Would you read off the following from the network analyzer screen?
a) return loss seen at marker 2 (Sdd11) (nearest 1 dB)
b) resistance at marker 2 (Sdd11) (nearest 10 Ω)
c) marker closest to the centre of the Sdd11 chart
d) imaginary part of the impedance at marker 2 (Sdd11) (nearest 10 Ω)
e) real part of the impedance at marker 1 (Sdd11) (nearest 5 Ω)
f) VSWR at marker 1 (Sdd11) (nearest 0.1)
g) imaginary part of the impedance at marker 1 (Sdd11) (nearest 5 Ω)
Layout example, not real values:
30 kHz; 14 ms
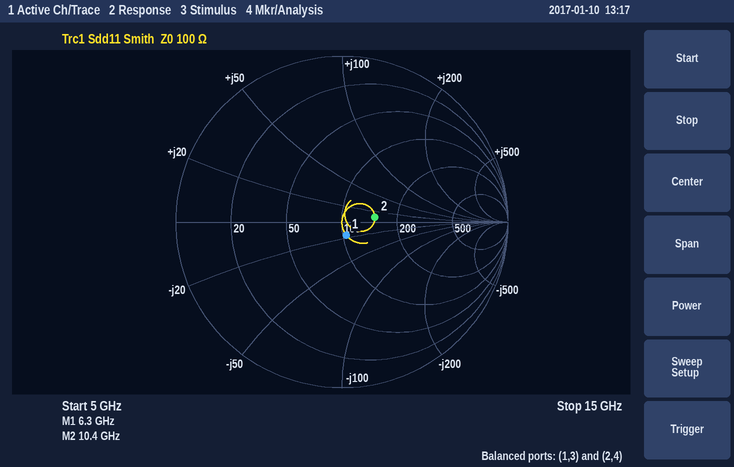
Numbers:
14 dB; 150 Ω; marker 1; +10 Ω; 105 Ω; 1.2; -15 Ω
